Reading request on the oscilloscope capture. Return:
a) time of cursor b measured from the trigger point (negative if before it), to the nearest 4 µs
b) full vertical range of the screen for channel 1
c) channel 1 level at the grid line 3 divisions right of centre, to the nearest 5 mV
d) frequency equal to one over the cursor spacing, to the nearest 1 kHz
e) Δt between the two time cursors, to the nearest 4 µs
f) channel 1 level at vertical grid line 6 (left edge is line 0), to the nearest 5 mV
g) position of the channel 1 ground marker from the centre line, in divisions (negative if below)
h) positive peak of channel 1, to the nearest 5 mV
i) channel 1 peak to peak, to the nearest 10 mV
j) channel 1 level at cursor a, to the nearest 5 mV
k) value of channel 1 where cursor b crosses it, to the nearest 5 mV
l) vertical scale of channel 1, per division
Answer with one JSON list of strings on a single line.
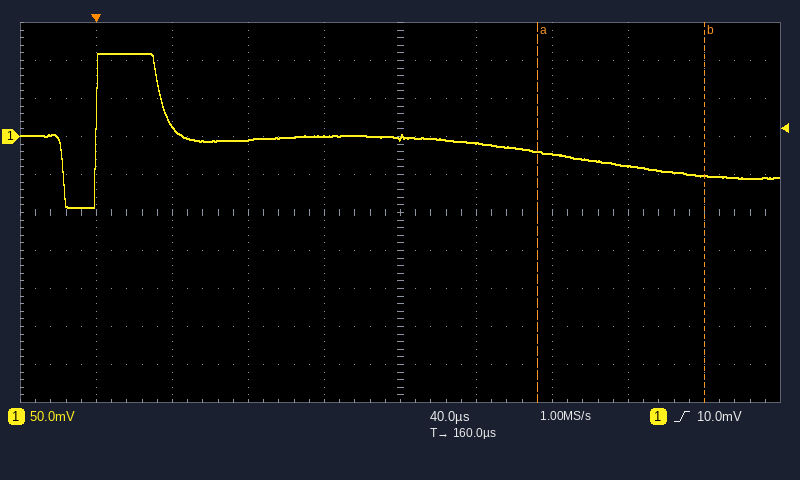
["+320 µs", "500 mV", "-40 mV", "11 kHz", "88 µs", "-10 mV", "+2.0 div", "110 mV", "200 mV", "-20 mV", "-50 mV", "50 mV"]
